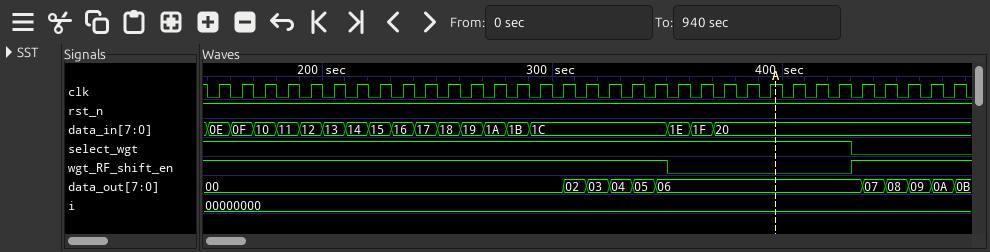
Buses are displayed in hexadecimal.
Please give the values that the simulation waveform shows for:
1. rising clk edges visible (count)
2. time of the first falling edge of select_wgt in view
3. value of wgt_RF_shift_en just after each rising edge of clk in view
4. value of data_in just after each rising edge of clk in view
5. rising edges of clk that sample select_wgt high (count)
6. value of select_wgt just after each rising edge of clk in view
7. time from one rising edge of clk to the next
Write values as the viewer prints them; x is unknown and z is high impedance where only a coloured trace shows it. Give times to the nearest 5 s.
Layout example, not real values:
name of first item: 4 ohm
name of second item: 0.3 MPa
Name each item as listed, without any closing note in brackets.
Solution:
rising clk edges visible: 33
time of the first falling edge of select_wgt in view: 430 s
value of wgt_RF_shift_en just after each rising edge of clk in view: 1 1 1 1 1 1 1 1 1 1 1 1 1 1 1 1 1 1 1 1 0 0 0 0 0 0 0 0 1 1 1 1 1
value of data_in just after each rising edge of clk in view: 0E, 0F, 10, 11, 12, 13, 14, 15, 16, 17, 18, 19, 1A, 1B, 1C, 1C, 1C, 1C, 1C, 1C, 1E, 1F, 20, 20, 20, 20, 20, 20, 20, 20, 20, 20, 20
rising edges of clk that sample select_wgt high: 28
value of select_wgt just after each rising edge of clk in view: 1 1 1 1 1 1 1 1 1 1 1 1 1 1 1 1 1 1 1 1 1 1 1 1 1 1 1 1 0 0 0 0 0
time from one rising edge of clk to the next: 10 s
